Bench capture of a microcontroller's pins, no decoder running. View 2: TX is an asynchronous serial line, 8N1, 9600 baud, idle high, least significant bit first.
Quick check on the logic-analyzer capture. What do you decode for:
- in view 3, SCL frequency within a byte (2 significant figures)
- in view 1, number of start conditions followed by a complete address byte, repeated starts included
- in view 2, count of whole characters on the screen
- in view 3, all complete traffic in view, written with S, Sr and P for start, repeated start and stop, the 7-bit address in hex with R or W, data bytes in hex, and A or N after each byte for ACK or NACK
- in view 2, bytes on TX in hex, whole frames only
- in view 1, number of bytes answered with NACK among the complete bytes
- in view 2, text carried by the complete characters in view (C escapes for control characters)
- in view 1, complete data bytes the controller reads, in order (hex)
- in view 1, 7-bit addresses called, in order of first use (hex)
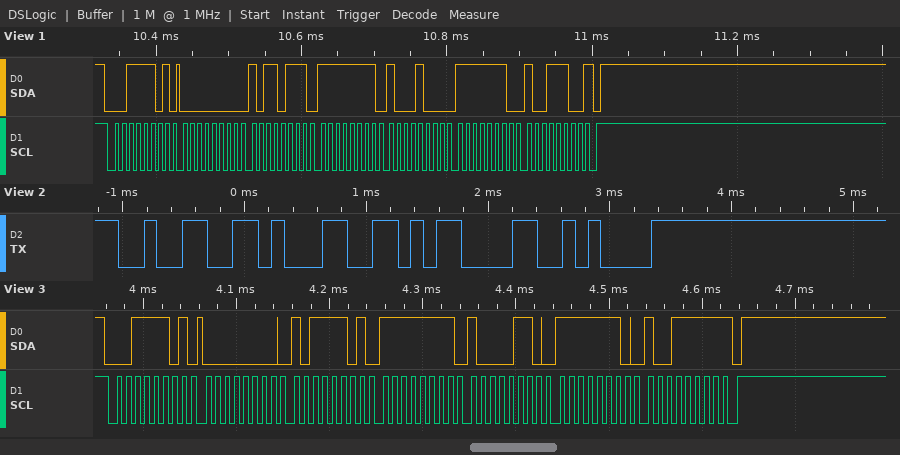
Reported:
100 kHz
1
4
S 1ER A 00 A BD A FF A 86 A FE A 9F N P
0x32 0x31 0x0D 0x0A
1
"21\r\n"
00 B7 FF 88 FE 9C
0x1E
